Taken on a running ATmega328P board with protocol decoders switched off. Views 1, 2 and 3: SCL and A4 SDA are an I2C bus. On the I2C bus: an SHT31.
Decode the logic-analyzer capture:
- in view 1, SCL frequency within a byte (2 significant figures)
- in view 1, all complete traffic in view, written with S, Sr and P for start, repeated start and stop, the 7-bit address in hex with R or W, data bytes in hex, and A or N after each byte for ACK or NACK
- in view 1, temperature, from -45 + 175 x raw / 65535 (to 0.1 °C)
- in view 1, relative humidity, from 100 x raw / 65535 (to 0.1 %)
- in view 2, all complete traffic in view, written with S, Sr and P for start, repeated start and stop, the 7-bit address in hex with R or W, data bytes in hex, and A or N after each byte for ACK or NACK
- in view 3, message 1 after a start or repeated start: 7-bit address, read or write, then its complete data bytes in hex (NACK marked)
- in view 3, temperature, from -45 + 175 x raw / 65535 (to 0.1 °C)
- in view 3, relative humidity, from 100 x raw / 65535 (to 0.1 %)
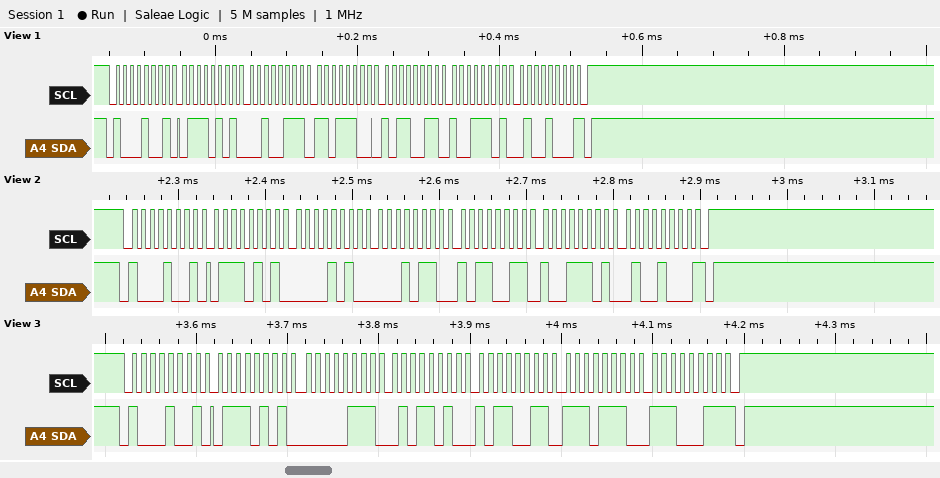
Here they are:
100 kHz
S 44R A 75 A 27 A DC A B3 A 9D A 48 N P
35.1 °C
70.2 %
S 44R A 75 A 0A A 16 A B3 A 9D A 48 N P
0x44 read: 75 07 5A B3 EE E3 NACK
35.0 °C
70.3 %
